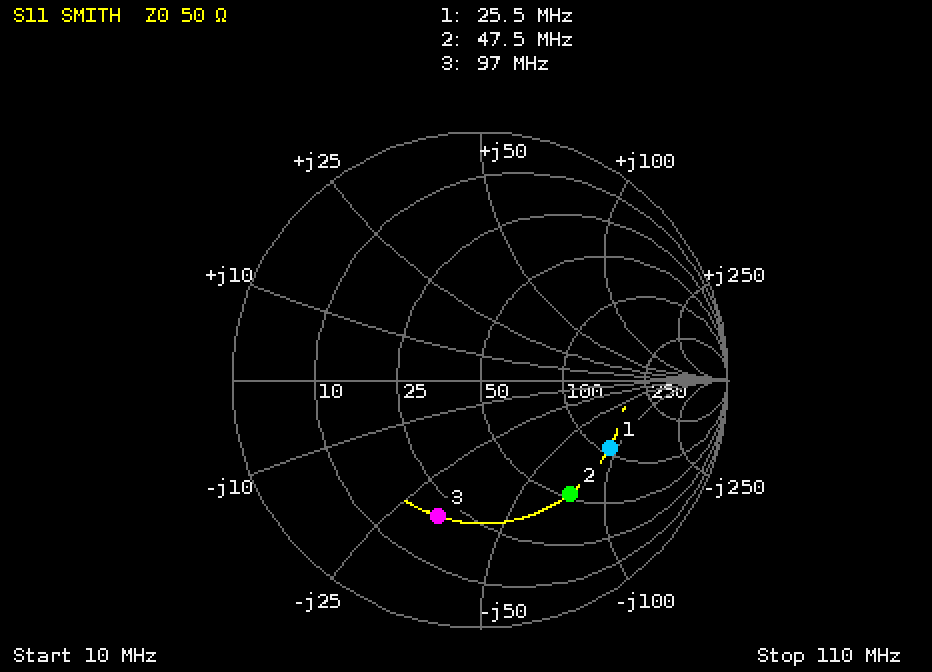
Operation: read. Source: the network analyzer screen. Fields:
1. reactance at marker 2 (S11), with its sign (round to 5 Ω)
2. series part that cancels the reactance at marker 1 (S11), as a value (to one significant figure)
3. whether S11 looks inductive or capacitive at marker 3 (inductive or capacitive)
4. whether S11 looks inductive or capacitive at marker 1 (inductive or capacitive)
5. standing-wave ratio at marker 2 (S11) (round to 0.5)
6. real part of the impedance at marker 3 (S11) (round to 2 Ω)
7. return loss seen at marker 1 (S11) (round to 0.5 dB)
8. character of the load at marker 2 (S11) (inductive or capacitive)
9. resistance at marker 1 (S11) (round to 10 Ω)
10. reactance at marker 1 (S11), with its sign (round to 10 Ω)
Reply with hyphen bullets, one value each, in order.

- -75 Ω
- 600 nH
- capacitive
- capacitive
- 4.0
- 20 Ω
- 4.5 dB
- capacitive
- 110 Ω
- -90 Ω
